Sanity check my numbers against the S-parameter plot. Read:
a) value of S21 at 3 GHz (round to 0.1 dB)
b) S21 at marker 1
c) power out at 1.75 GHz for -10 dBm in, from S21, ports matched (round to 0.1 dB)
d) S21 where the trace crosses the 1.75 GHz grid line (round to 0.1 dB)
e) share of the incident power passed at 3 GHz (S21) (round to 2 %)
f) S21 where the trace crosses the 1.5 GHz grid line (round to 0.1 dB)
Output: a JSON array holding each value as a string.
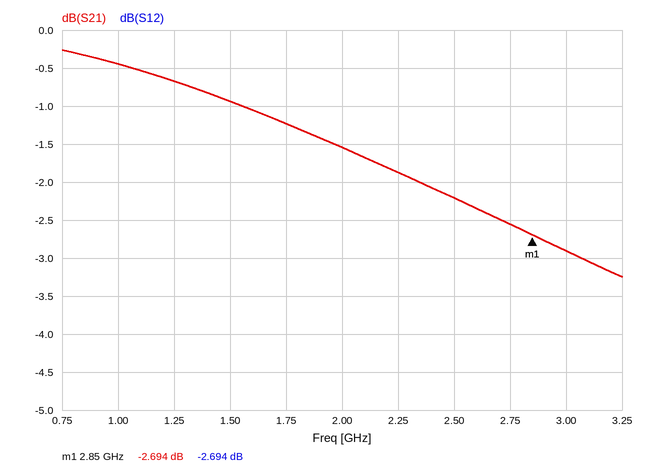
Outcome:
["-2.9 dB", "-2.694 dB", "-11.2 dBm", "-1.2 dB", "52 %", "-0.9 dB"]
